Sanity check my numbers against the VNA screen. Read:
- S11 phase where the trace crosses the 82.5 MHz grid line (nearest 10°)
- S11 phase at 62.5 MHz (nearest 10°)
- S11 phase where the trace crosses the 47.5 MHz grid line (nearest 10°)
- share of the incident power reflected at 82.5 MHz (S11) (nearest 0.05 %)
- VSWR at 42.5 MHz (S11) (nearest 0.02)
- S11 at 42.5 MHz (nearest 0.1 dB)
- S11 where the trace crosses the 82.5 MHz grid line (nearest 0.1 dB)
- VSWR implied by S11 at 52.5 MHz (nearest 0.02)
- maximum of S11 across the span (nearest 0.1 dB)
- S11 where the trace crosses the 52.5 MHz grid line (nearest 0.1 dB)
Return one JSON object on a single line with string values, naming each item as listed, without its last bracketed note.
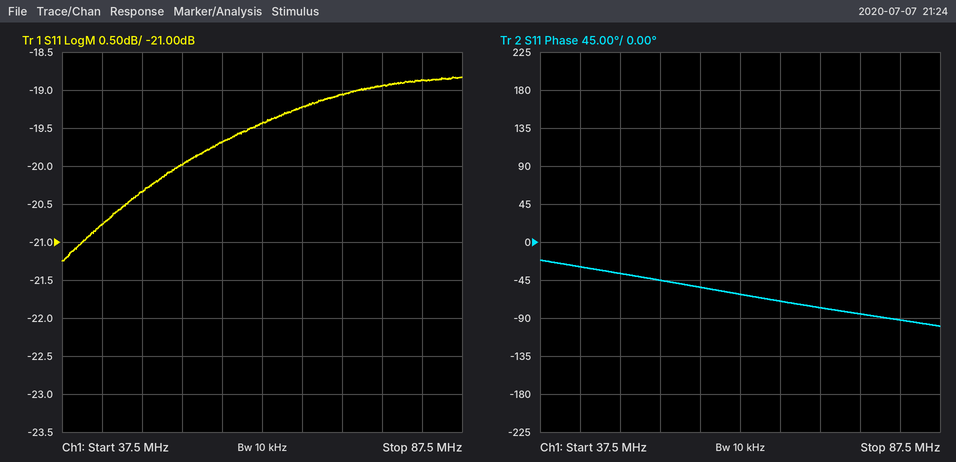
{"S11 phase where the trace crosses the 82.5 MHz grid line": "-90°", "S11 phase at 62.5 MHz": "-60°", "S11 phase where the trace crosses the 47.5 MHz grid line": "-40°", "share of the incident power reflected at 82.5 MHz (S11)": "1.30 %", "VSWR at 42.5 MHz (S11)": "1.20", "S11 at 42.5 MHz": "-20.8 dB", "S11 where the trace crosses the 82.5 MHz grid line": "-18.9 dB", "VSWR implied by S11 at 52.5 MHz": "1.22", "maximum of S11 across the span": "-18.8 dB", "S11 where the trace crosses the 52.5 MHz grid line": "-20.0 dB"}
